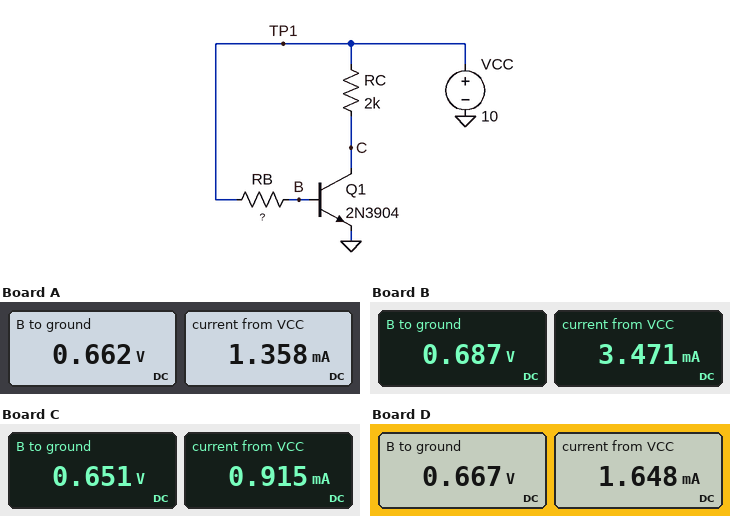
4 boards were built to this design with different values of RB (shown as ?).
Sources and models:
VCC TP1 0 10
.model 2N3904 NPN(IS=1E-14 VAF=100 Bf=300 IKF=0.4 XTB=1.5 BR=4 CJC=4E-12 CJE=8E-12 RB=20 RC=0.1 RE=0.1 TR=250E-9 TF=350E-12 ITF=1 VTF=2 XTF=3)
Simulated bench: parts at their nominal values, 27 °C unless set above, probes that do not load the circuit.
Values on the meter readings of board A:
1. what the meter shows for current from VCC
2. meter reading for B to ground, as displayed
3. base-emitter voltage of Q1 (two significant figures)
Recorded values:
1.358 mA
0.662 V
660 mV
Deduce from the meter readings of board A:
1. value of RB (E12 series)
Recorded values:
2.2 MΩ
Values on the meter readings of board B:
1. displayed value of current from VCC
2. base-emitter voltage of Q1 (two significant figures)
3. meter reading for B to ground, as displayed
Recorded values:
3.471 mA
690 mV
0.687 V
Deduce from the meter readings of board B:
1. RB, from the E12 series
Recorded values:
820 kΩ
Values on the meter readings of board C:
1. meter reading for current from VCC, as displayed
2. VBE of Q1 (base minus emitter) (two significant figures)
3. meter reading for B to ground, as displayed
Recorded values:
0.915 mA
650 mV
0.651 V
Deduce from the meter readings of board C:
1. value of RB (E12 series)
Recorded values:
3.3 MΩ
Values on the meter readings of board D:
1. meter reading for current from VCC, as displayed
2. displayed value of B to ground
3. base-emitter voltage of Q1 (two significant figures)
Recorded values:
1.648 mA
0.667 V
670 mV
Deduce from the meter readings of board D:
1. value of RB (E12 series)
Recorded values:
1.8 MΩ
